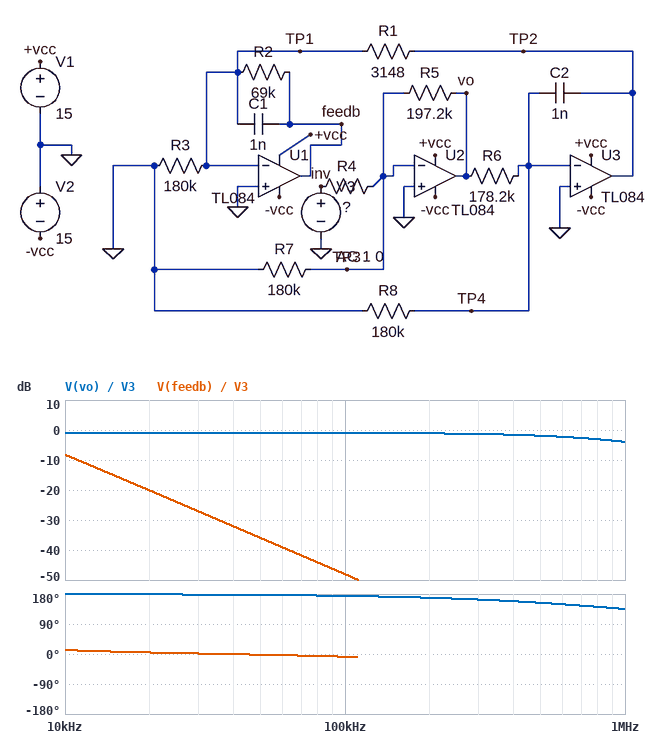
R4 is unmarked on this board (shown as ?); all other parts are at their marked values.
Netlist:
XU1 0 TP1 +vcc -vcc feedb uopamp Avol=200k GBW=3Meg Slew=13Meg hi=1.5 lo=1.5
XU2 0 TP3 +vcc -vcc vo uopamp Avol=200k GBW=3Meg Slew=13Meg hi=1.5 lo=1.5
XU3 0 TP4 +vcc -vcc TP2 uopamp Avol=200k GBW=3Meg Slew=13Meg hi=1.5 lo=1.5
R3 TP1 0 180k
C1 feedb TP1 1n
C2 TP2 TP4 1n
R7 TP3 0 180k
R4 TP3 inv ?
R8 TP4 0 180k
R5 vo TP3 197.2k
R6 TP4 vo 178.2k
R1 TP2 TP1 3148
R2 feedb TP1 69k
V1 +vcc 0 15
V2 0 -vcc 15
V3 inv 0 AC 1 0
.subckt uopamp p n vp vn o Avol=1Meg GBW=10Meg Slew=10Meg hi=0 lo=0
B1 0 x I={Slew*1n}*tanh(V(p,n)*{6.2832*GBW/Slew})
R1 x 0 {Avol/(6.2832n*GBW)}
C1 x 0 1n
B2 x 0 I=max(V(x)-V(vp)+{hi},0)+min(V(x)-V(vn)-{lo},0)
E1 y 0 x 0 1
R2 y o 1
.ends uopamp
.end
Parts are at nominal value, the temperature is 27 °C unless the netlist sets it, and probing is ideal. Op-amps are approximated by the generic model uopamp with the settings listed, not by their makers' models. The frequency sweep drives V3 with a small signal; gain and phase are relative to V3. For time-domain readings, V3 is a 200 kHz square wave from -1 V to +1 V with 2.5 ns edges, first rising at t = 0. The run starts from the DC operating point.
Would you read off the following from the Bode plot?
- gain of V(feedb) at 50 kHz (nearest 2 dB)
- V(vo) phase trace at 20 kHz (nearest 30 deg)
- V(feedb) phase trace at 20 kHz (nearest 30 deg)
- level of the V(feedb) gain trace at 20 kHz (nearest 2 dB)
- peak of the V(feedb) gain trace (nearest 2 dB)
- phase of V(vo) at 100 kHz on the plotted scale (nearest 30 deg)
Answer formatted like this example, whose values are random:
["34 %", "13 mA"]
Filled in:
["-36 dB", "180 deg", "0 deg", "-20 dB", "-8 dB", "180 deg"]
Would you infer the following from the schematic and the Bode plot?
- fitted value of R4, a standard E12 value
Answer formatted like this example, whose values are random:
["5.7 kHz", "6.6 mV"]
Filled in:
["220 kΩ"]
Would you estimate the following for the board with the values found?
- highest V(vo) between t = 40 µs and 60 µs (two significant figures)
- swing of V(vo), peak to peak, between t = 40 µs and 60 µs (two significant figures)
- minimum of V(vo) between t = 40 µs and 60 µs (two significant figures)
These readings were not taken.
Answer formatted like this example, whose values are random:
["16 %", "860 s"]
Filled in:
["900 mV", "1.8 V", "-900 mV"]
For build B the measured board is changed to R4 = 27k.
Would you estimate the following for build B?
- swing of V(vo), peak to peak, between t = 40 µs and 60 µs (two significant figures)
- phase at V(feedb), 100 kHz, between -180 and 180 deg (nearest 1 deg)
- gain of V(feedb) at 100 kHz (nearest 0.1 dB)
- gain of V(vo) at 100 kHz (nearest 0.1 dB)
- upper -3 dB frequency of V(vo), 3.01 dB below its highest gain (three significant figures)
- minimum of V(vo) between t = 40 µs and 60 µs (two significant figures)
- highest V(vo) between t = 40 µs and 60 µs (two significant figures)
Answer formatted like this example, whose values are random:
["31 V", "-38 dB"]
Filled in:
["14 V", "-20 deg", "-30.2 dB", "16.9 dB", "319 kHz", "-7.1 V", "7.1 V"]
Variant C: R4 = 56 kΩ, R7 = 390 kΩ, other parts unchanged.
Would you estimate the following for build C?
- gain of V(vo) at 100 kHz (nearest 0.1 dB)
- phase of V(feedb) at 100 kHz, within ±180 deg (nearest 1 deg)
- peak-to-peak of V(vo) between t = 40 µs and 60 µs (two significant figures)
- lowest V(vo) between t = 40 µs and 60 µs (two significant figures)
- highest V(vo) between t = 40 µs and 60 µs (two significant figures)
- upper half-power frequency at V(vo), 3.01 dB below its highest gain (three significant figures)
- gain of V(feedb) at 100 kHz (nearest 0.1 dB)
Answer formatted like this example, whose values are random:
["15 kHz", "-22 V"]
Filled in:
["10.8 dB", "-12 deg", "7.0 V", "-3.5 V", "3.5 V", "597 kHz", "-36.3 dB"]
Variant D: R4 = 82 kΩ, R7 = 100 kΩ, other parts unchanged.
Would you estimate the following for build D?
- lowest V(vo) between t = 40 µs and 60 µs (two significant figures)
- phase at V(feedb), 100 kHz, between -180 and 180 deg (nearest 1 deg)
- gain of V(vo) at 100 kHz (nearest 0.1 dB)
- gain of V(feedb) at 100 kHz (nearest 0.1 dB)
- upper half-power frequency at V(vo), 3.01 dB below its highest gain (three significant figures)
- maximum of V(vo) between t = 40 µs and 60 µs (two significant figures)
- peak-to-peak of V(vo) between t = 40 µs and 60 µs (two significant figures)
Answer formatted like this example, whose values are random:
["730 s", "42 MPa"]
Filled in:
["-2.4 V", "-13 deg", "7.5 dB", "-39.6 dB", "558 kHz", "2.4 V", "4.8 V"]
